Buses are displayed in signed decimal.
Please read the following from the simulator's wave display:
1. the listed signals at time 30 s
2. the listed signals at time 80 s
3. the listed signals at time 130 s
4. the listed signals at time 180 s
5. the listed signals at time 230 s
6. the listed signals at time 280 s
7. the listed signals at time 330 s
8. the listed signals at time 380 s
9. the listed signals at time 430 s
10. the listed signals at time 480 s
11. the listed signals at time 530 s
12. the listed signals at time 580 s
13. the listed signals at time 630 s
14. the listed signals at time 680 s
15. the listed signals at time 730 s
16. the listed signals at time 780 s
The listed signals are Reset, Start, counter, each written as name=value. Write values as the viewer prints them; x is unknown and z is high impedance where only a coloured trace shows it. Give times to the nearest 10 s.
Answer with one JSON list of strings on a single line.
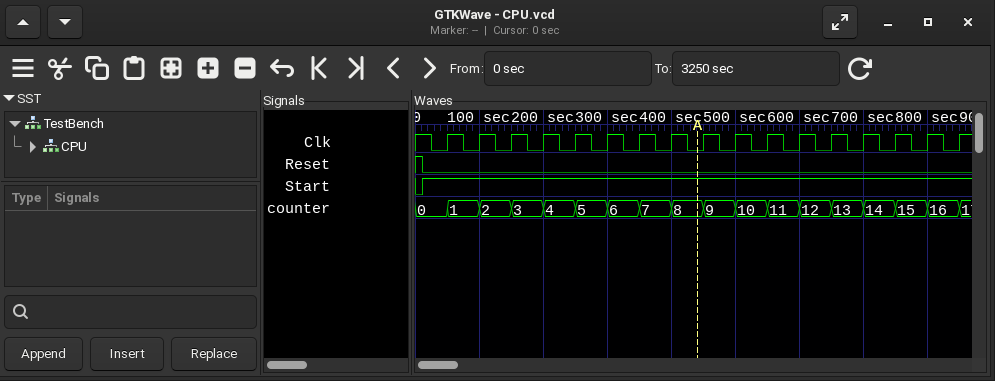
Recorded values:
["Reset=0, Start=1, counter=0", "Reset=0, Start=1, counter=1", "Reset=0, Start=1, counter=2", "Reset=0, Start=1, counter=3", "Reset=0, Start=1, counter=4", "Reset=0, Start=1, counter=5", "Reset=0, Start=1, counter=6", "Reset=0, Start=1, counter=7", "Reset=0, Start=1, counter=8", "Reset=0, Start=1, counter=9", "Reset=0, Start=1, counter=10", "Reset=0, Start=1, counter=11", "Reset=0, Start=1, counter=12", "Reset=0, Start=1, counter=13", "Reset=0, Start=1, counter=14", "Reset=0, Start=1, counter=15"]
